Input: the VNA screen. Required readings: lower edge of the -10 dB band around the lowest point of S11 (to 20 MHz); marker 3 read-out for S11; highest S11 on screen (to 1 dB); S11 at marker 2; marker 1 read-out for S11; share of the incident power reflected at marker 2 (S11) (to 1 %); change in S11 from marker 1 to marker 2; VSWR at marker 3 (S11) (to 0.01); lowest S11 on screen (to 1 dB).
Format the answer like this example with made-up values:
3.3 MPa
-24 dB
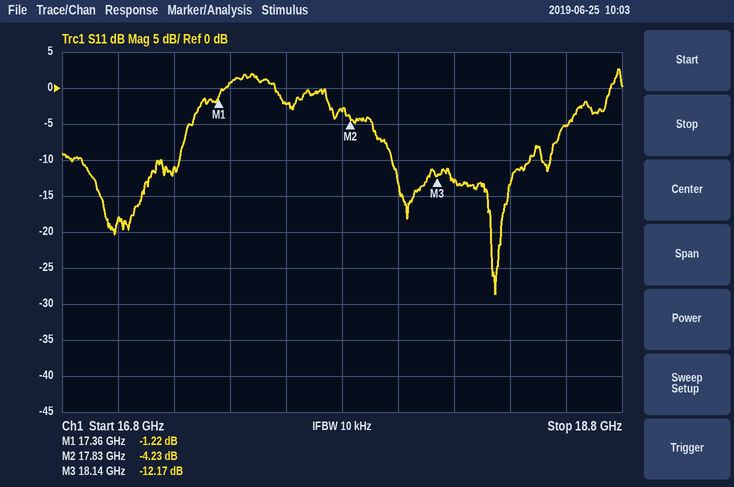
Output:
17.98 GHz
-12.17 dB
3 dB
-4.23 dB
-1.22 dB
38 %
-3.01 dB
1.65
-29 dB
